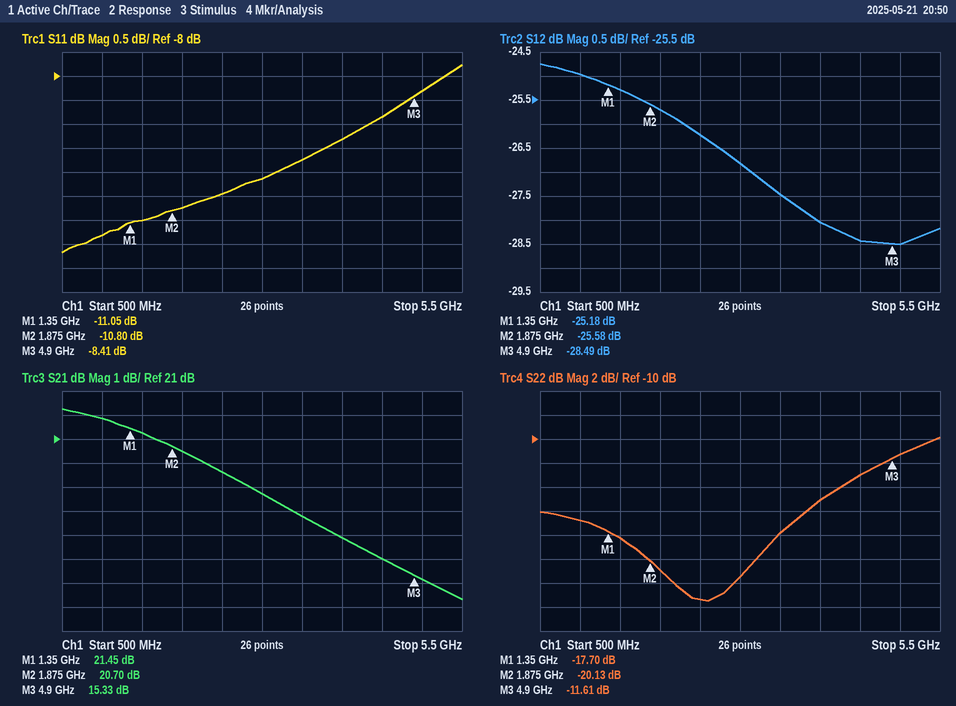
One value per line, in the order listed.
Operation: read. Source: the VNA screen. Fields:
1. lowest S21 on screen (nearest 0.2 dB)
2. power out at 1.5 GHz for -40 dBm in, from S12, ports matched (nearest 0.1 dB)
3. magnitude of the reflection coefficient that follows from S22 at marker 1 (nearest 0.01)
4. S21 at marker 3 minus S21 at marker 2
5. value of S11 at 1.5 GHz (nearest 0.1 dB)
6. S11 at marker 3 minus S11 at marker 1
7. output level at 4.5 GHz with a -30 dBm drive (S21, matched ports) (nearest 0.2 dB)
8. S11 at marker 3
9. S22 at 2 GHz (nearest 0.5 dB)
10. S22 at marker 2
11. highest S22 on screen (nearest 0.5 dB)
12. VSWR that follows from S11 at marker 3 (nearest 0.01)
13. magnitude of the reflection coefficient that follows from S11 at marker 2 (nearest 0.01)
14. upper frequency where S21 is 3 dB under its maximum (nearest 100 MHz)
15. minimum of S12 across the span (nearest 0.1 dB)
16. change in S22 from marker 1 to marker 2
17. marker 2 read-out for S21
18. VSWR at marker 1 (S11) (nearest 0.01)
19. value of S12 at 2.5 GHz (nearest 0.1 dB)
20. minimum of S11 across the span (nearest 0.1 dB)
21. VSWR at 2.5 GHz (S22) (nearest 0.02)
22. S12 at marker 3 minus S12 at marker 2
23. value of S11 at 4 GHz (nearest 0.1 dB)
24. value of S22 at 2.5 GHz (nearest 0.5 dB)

14.4 dB
-65.3 dBm
0.13
-5.37 dB
-11.0 dB
2.64 dB
-14.0 dBm
-8.41 dB
-21.0 dB
-20.13 dB
-10.0 dB
2.22
0.29
2.7 GHz
-28.5 dB
-2.43 dB
20.70 dB
1.78
-26.2 dB
-11.7 dB
1.14
-2.91 dB
-9.3 dB
-23.5 dB
